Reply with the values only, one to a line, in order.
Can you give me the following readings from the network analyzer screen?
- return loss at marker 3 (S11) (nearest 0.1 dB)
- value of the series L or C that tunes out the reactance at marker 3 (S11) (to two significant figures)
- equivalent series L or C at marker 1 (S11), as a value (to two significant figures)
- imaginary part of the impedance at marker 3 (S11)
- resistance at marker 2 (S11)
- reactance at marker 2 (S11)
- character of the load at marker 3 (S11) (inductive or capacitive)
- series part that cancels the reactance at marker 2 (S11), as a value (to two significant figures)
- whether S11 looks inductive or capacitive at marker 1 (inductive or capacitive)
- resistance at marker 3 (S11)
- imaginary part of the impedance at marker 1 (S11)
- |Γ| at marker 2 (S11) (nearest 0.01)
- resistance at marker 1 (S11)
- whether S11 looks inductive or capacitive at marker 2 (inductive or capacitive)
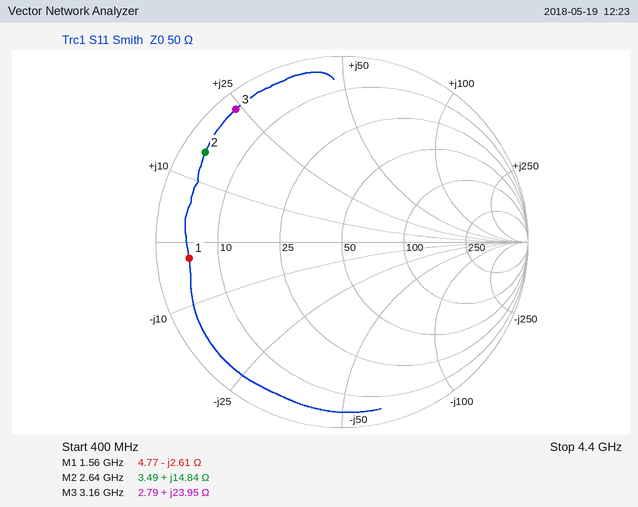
0.8 dB
2.1 pF
39 pF
+23.95 Ω
3.49 Ω
+14.84 Ω
inductive
4.1 pF
capacitive
2.79 Ω
-2.61 Ω
0.88
4.77 Ω
inductive
